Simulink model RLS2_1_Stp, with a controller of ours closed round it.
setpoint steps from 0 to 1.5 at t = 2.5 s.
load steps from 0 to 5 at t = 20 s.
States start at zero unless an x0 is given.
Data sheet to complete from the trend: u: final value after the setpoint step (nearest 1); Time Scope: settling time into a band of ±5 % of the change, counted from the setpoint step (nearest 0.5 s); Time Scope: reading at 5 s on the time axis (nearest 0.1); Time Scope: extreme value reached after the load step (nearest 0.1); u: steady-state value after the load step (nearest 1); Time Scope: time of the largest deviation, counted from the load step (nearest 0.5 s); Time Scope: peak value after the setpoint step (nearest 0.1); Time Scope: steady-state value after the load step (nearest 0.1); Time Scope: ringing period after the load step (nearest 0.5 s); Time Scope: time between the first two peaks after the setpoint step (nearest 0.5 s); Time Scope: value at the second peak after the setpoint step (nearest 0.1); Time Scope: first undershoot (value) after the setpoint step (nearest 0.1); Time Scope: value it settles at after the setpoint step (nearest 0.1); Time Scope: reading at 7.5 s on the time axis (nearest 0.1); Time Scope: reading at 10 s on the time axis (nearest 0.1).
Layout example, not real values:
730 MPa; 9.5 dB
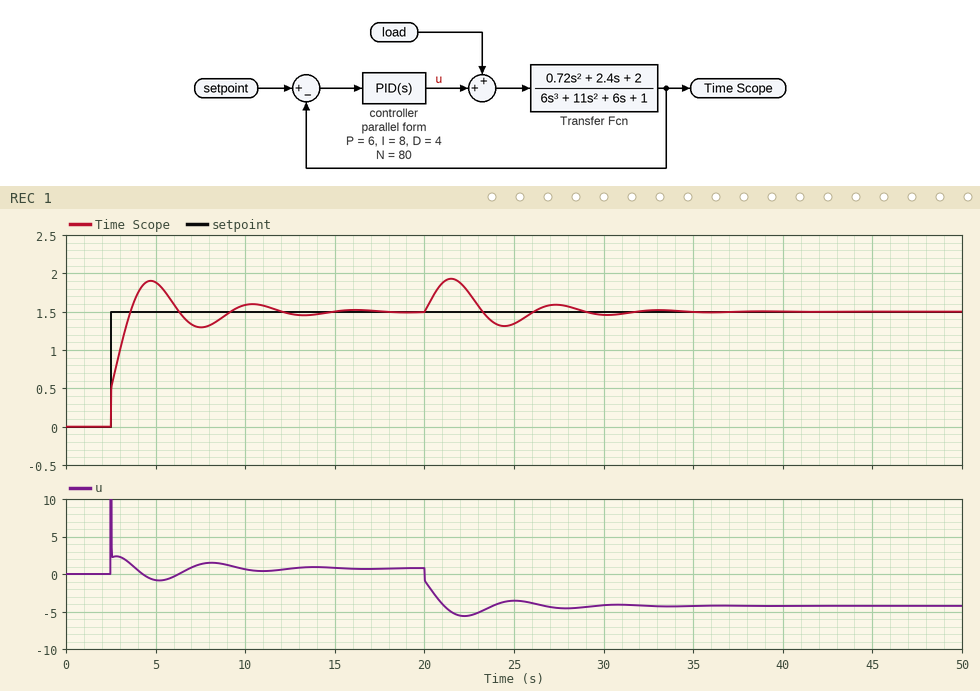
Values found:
1; 8.5 s; 1.9; 1.9; -4; 1.5 s; 1.9; 1.5; 6.0 s; 5.5 s; 1.6; 1.3; 1.5; 1.3; 1.6
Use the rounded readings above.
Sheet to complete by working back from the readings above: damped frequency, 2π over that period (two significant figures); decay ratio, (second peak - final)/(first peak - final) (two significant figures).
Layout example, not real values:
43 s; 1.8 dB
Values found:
1.1 rad/s; 0.25
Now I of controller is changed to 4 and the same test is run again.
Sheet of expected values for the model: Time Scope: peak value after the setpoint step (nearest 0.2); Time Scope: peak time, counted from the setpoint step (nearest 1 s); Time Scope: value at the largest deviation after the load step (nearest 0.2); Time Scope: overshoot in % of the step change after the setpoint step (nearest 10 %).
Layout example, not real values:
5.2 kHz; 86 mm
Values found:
1.8; 3 s; 2.0; 20 %
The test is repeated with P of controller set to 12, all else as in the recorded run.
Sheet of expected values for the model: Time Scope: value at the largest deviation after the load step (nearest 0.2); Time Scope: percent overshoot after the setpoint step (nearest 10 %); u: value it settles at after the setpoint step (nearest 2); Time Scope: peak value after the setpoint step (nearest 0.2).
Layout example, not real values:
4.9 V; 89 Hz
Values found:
1.8; 20 %; 0; 1.8
